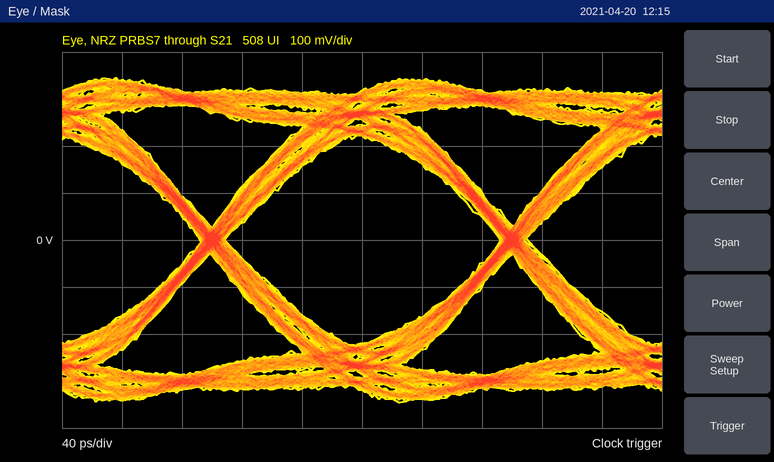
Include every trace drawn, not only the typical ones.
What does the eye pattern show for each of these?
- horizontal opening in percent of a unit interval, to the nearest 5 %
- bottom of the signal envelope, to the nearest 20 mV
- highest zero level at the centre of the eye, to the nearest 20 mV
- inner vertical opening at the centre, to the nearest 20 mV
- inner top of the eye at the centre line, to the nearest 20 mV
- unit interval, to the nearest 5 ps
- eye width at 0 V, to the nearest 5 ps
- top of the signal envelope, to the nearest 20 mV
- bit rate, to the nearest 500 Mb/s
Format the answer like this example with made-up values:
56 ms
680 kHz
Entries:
90 %
-340 mV
-220 mV
440 mV
220 mV
200 ps
185 ps
340 mV
5.0 Gb/s
